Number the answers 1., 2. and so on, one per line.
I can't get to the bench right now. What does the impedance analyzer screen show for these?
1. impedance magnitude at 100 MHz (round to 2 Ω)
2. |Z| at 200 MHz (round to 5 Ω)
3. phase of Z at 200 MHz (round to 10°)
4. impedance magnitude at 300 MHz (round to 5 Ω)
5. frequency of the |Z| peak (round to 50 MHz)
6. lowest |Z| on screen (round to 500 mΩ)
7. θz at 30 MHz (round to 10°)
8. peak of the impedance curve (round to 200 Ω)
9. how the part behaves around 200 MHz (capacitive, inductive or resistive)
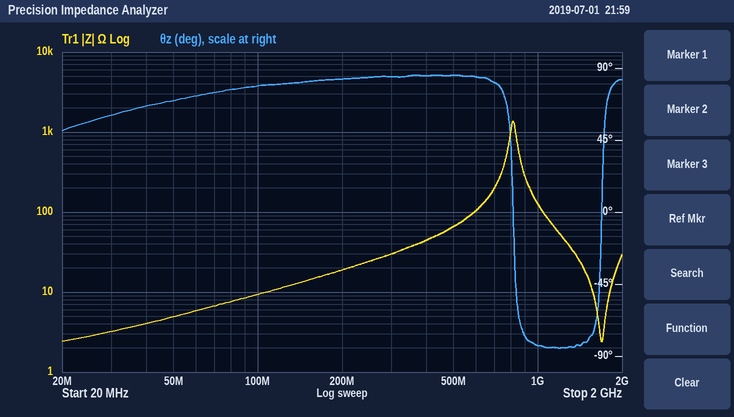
1. 10 Ω
2. 20 Ω
3. 80°
4. 30 Ω
5. 800 MHz
6. 2.5 Ω
7. 60°
8. 1.4 kΩ
9. inductive
